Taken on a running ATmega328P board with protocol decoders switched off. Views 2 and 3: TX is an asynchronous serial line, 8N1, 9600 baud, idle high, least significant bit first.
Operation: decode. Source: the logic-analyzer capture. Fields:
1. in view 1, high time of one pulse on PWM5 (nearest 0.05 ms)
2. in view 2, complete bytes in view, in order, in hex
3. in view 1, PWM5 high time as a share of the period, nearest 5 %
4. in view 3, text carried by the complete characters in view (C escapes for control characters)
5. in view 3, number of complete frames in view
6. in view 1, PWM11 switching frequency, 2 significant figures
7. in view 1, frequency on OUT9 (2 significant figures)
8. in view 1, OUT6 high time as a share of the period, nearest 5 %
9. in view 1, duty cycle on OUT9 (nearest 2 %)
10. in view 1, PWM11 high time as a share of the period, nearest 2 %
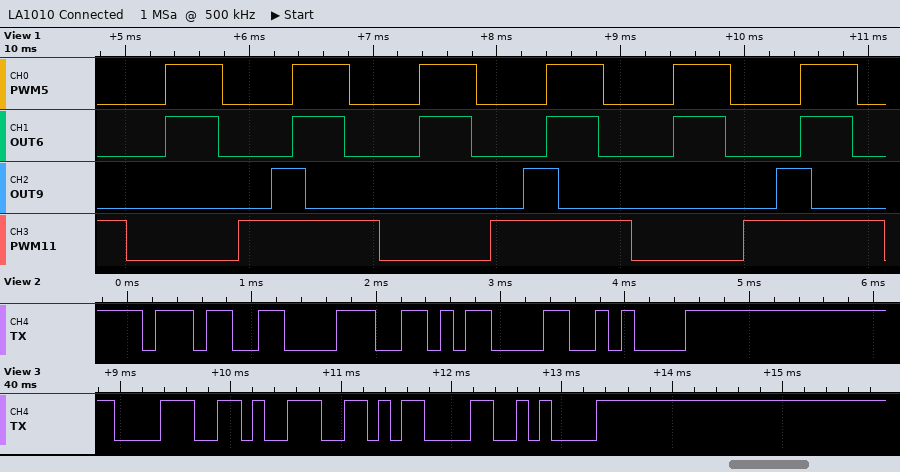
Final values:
0.45 ms
37 38 0D 0A
45 %
"89\r\n"
4
490 Hz
490 Hz
40 %
14 %
56 %
